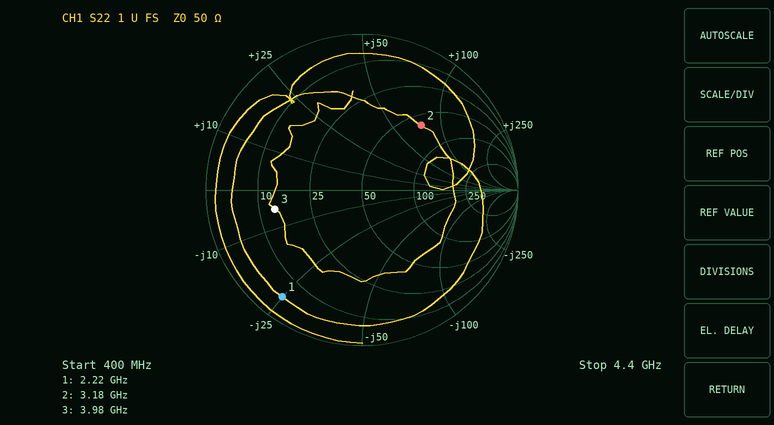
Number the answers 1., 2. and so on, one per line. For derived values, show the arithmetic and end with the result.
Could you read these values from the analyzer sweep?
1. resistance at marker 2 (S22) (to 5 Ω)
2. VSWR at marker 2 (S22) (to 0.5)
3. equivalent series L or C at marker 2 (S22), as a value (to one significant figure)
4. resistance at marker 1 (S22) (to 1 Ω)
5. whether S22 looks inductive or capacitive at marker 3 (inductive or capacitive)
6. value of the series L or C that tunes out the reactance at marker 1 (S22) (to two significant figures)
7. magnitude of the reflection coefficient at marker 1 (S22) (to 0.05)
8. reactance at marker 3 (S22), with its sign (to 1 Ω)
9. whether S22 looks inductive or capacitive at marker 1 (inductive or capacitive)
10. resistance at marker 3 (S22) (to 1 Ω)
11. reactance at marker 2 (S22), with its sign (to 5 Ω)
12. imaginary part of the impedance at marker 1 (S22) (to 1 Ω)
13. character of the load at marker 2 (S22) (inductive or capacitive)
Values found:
1. 60 Ω
2. 3.5
3. L = 75 Ω/(2π × 3.18 GHz) ≈ 4 nH
4. 5 Ω
5. capacitive
6. L = 25 Ω/(2π × 2.22 GHz) ≈ 1.8 nH
7. 0.85
8. -5 Ω
9. capacitive
10. 14 Ω
11. +75 Ω
12. -25 Ω
13. inductive
